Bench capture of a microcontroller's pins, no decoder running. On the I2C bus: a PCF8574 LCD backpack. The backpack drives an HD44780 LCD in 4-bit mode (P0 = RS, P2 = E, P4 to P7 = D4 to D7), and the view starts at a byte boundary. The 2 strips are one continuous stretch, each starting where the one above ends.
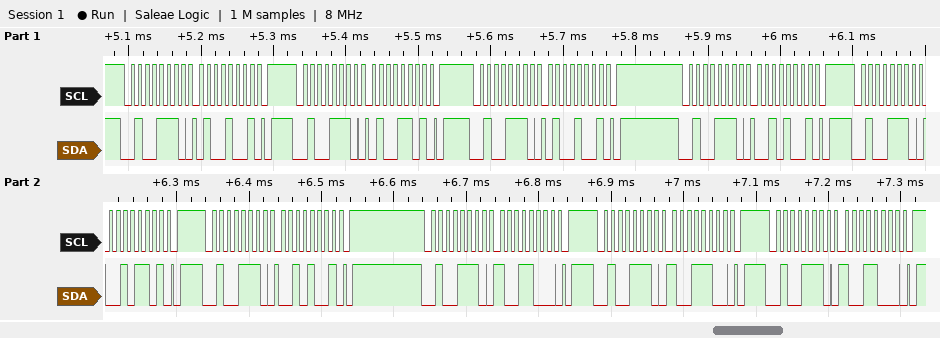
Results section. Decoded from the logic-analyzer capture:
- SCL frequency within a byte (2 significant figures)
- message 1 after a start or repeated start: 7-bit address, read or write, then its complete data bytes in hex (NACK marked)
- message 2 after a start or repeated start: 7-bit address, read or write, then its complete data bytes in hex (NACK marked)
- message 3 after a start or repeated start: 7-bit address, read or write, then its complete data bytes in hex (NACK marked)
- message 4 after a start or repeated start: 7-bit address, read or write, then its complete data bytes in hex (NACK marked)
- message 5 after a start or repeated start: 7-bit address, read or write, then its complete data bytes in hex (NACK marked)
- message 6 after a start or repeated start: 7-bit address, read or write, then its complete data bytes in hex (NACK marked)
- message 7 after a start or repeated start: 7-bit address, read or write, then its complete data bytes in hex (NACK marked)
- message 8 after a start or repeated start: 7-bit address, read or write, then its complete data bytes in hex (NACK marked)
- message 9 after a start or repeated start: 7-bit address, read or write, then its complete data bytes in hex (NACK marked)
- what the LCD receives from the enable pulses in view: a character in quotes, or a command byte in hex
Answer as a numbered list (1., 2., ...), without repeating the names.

1. 100 kHz
2. 0x27 write: 49
3. 0x27 write: 4D
4. 0x27 write: 49
5. 0x27 write: 29
6. 0x27 write: 2D
7. 0x27 write: 29
8. 0x27 write: 98
9. 0x27 write: 9C
10. 0x27 write: 98
11. 'B'
